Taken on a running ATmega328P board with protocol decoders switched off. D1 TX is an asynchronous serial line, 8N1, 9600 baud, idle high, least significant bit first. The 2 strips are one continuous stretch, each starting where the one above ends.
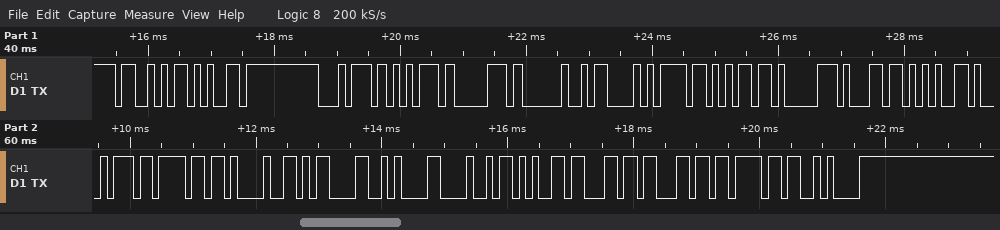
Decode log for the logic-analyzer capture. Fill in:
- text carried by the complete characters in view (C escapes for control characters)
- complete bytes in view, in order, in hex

"Setup Completo!\r\nHello\n"
53 65 74 75 70 20 43 6F 6D 70 6C 65 74 6F 21 0D 0A 48 65 6C 6C 6F 0A
